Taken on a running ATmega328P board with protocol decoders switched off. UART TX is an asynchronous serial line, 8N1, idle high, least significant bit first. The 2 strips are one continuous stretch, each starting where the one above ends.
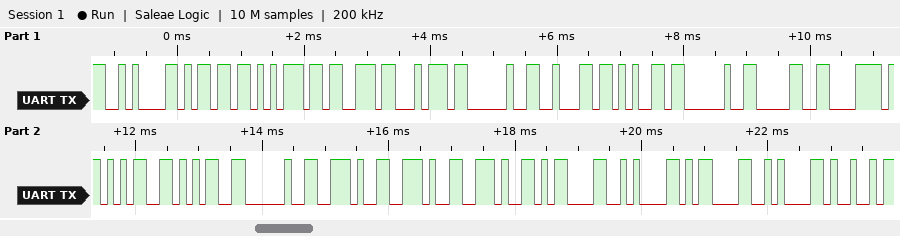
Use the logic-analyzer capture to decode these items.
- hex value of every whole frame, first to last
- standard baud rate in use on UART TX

0x0A 0x6D 0x75 0x73 0x74 0x20 0x62 0x65 0x20 0x30 0x78 0x35 0x35 0x20 0x2E 0x2E 0x2E 0x0D 0x0A 0x0D 0x0A 0x49
9600 baud
